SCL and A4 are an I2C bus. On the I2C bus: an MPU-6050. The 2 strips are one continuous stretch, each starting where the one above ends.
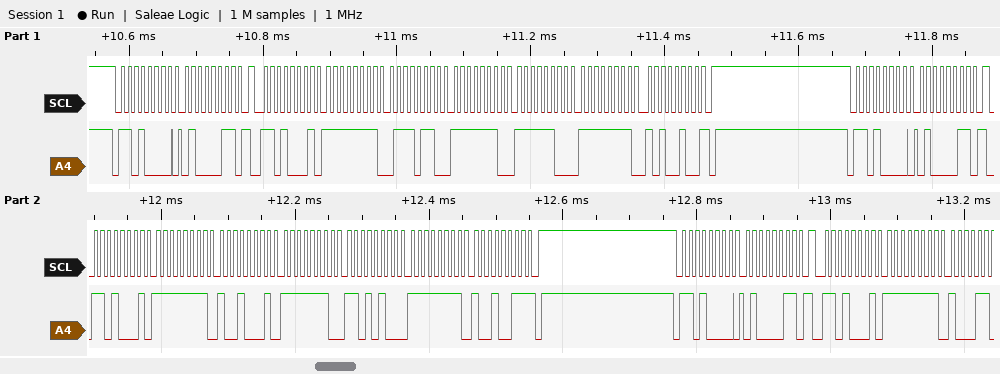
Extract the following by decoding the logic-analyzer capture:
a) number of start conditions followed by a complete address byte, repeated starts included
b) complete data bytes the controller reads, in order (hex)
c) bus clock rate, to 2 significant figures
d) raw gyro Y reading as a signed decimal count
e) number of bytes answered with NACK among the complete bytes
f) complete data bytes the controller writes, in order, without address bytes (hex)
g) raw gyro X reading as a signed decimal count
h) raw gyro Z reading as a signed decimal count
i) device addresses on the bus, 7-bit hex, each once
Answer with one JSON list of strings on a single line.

["6", "FF 76 FE FC FF A4 FF 91 FE D4 FF 93 FF", "100 kHz", "-260", "2", "43 43 43", "-138", "-92", "0x68"]
